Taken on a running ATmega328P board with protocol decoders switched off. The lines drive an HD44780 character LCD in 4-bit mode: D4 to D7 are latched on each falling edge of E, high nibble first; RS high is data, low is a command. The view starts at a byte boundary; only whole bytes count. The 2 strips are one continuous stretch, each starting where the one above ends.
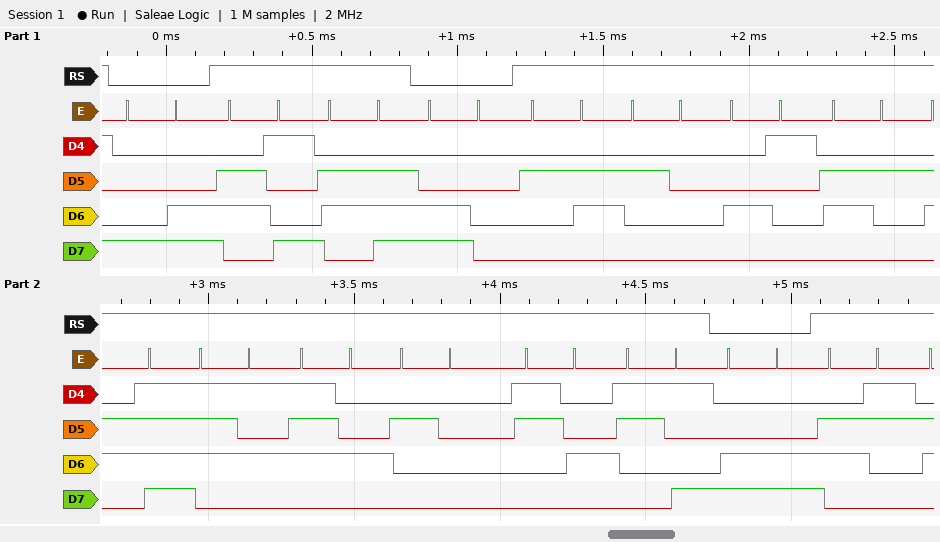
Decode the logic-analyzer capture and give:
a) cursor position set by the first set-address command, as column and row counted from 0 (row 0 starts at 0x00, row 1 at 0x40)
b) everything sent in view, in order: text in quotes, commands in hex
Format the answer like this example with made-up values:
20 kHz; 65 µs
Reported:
column 12, row 0; 0x8C "in" 0xC0 "& About 49" 0xCC "c"
